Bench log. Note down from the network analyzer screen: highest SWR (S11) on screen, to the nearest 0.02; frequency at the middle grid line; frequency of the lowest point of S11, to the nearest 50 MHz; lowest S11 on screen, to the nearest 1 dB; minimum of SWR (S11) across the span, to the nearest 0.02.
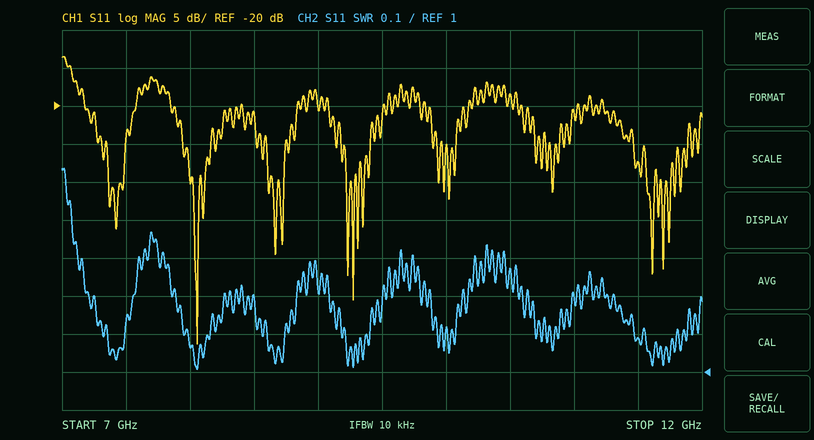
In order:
1.54
9.5 GHz
8.05 GHz
-51 dB
1.00
